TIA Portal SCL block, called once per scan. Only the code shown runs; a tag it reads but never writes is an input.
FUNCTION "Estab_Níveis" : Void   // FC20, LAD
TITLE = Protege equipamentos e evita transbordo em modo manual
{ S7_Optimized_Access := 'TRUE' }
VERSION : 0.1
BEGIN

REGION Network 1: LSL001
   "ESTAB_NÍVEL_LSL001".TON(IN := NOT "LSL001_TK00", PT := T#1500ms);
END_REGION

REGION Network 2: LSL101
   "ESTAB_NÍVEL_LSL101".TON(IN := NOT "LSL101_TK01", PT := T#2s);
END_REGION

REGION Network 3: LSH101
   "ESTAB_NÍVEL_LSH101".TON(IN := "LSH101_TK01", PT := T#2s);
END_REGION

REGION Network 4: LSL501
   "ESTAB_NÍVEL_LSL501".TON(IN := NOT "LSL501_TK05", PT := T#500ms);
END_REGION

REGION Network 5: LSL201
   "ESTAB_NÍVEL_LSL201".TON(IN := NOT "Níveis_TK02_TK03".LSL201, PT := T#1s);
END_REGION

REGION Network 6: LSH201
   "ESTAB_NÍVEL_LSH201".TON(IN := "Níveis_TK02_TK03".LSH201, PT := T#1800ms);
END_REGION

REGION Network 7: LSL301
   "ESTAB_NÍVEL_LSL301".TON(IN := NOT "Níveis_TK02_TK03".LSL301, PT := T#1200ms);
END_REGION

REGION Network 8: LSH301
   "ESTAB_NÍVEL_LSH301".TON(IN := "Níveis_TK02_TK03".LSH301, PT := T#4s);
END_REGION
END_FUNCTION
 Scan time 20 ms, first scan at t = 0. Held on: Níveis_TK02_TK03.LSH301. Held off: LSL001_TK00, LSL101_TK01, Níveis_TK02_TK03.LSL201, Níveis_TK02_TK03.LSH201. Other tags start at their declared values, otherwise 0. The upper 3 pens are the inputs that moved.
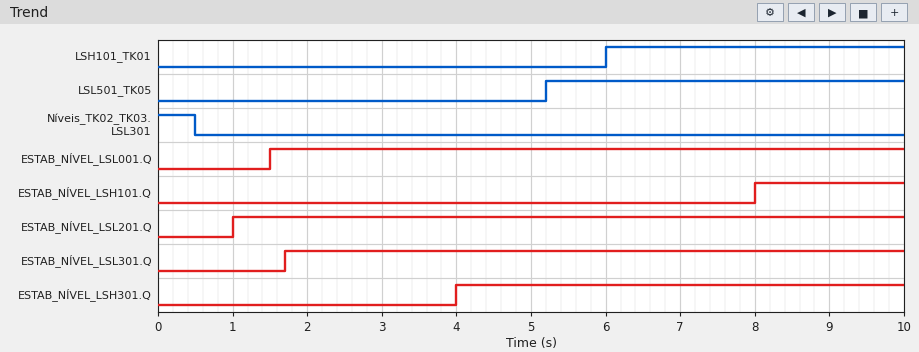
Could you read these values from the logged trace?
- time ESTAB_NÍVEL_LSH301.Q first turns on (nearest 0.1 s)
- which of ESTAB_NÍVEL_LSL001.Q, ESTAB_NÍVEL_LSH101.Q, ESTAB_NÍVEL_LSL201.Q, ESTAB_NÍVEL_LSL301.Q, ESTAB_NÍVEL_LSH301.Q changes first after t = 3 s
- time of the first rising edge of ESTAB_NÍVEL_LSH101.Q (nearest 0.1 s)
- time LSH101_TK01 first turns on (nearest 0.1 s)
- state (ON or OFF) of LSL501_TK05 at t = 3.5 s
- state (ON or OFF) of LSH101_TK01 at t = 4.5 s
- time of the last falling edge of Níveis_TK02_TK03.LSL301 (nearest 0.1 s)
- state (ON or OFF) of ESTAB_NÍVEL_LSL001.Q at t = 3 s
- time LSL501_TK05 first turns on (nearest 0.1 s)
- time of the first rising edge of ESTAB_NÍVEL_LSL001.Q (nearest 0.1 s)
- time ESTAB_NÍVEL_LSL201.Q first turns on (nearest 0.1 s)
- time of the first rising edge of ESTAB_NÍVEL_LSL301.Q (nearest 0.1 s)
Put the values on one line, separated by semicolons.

4.0 s; ESTAB_NÍVEL_LSH301.Q; 8.0 s; 6.0 s; OFF; OFF; 0.5 s; ON; 5.2 s; 1.5 s; 1.0 s; 1.7 s
